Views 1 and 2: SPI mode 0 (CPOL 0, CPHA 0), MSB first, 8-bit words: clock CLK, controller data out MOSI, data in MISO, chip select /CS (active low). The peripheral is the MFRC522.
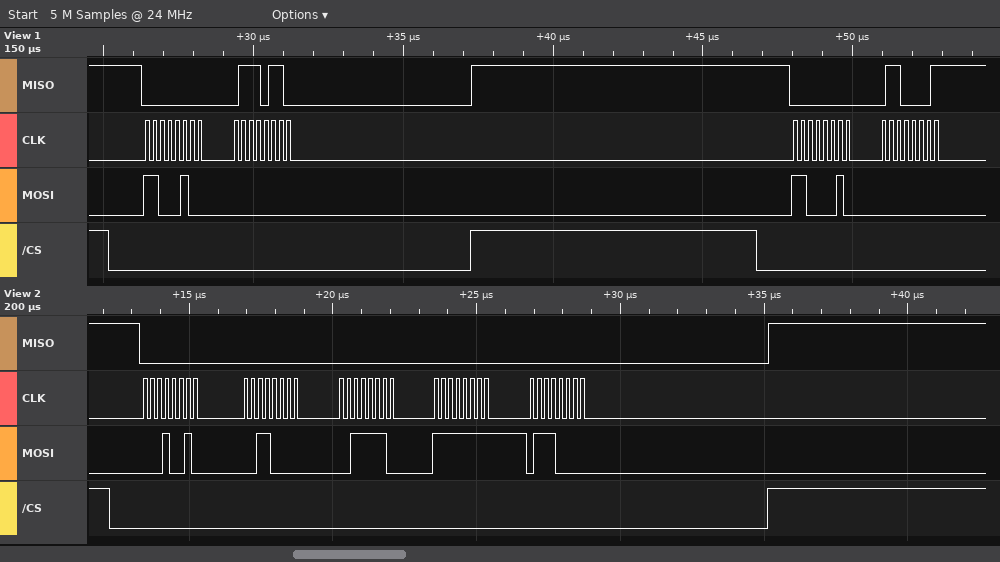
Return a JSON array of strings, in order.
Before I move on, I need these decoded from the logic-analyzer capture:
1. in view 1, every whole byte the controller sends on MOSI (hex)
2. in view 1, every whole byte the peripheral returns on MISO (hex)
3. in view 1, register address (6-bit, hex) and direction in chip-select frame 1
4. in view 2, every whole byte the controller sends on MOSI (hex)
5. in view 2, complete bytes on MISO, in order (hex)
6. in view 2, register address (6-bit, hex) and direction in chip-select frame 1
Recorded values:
["C4 00 C2 00", "00 76 00 61", "0x22 read", "12 30 3E FF 70", "00 00 00 00 00", "0x09 write"]
